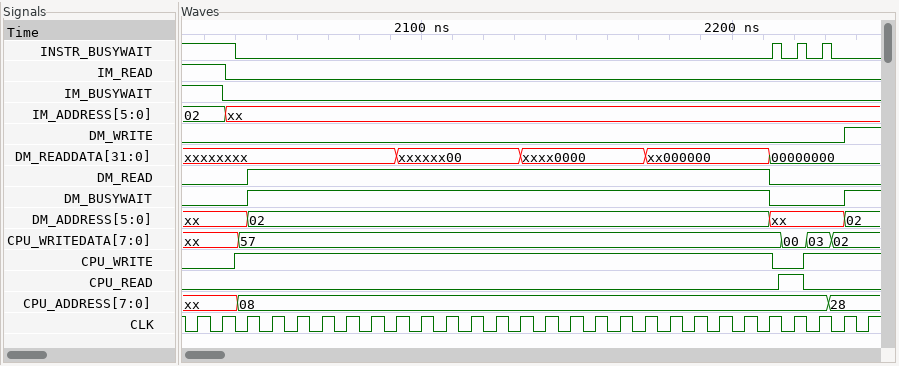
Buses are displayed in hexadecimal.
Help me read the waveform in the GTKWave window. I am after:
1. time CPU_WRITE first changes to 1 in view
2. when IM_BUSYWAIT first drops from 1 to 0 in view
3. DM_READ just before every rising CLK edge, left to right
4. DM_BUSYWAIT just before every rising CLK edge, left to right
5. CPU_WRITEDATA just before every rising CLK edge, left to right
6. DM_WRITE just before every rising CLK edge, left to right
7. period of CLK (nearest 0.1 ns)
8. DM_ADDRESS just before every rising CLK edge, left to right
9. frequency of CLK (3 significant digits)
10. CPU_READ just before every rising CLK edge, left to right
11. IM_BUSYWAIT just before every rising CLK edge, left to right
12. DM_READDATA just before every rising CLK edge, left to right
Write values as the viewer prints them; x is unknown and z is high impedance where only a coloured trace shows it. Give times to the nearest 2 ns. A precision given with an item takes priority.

2040 ns
2036 ns
0 0 0 1 1 1 1 1 1 1 1 1 1 1 1 1 1 1 1 1 1 1 1 1 0 0 0 0
0 0 0 1 1 1 1 1 1 1 1 1 1 1 1 1 1 1 1 1 1 1 1 1 0 0 0 1
xx, xx, 57, 57, 57, 57, 57, 57, 57, 57, 57, 57, 57, 57, 57, 57, 57, 57, 57, 57, 57, 57, 57, 57, 00, 03, 02, 02
0 0 0 0 0 0 0 0 0 0 0 0 0 0 0 0 0 0 0 0 0 0 0 0 0 0 0 1
8 ns
xx, xx, xx, 02, 02, 02, 02, 02, 02, 02, 02, 02, 02, 02, 02, 02, 02, 02, 02, 02, 02, 02, 02, 02, xx, xx, xx, 02
125 MHz
0 0 0 0 0 0 0 0 0 0 0 0 0 0 0 0 0 0 0 0 0 0 0 0 1 0 0 0
1 1 0 0 0 0 0 0 0 0 0 0 0 0 0 0 0 0 0 0 0 0 0 0 0 0 0 0
xxxxxxxx, xxxxxxxx, xxxxxxxx, xxxxxxxx, xxxxxxxx, xxxxxxxx, xxxxxxxx, xxxxxxxx, xxxxxxxx, xxxxxx00, xxxxxx00, xxxxxx00, xxxxxx00, xxxxxx00, xxxx0000, xxxx0000, xxxx0000, xxxx0000, xxxx0000, xx000000, xx000000, xx000000, xx000000, xx000000, 00000000, 00000000, 00000000, 00000000
